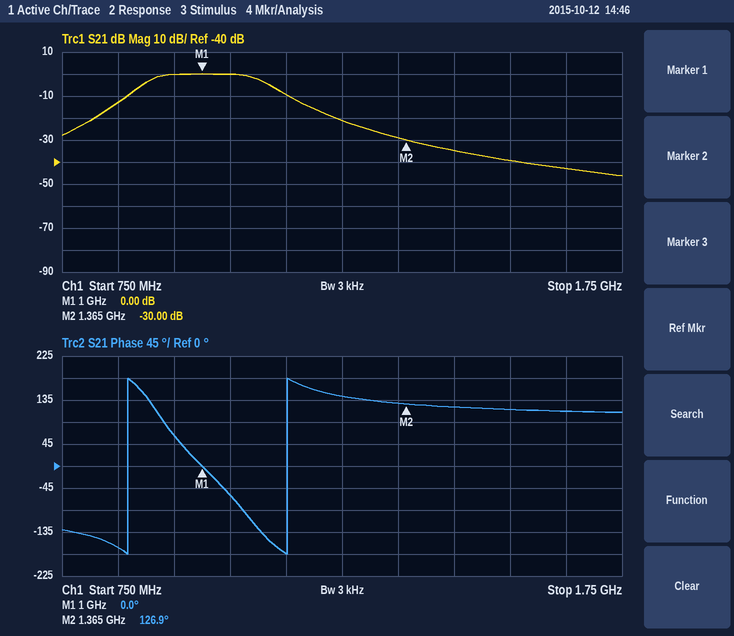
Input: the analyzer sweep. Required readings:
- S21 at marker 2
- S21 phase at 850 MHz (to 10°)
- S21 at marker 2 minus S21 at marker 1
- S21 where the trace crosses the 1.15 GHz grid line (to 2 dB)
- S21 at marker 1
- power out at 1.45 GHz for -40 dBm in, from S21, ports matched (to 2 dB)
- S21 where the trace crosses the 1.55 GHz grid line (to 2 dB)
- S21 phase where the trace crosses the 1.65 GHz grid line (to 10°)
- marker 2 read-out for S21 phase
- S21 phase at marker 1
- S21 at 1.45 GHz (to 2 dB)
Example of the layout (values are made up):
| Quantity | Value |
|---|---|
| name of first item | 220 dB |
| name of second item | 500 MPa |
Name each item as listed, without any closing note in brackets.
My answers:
| Quantity | Value |
|---|---|
| S21 at marker 2 | -30.00 dB |
| S21 phase at 850 MHz | -170° |
| S21 at marker 2 minus S21 at marker 1 | -30.00 dB |
| S21 where the trace crosses the 1.15 GHz grid line | -10 dB |
| S21 at marker 1 | 0.00 dB |
| power out at 1.45 GHz for -40 dBm in, from S21, ports matched | -74 dBm |
| S21 where the trace crosses the 1.55 GHz grid line | -40 dB |
| S21 phase where the trace crosses the 1.65 GHz grid line | 110° |
| marker 2 read-out for S21 phase | 126.9° |
| S21 phase at marker 1 | 0.0° |
| S21 at 1.45 GHz | -34 dB |
